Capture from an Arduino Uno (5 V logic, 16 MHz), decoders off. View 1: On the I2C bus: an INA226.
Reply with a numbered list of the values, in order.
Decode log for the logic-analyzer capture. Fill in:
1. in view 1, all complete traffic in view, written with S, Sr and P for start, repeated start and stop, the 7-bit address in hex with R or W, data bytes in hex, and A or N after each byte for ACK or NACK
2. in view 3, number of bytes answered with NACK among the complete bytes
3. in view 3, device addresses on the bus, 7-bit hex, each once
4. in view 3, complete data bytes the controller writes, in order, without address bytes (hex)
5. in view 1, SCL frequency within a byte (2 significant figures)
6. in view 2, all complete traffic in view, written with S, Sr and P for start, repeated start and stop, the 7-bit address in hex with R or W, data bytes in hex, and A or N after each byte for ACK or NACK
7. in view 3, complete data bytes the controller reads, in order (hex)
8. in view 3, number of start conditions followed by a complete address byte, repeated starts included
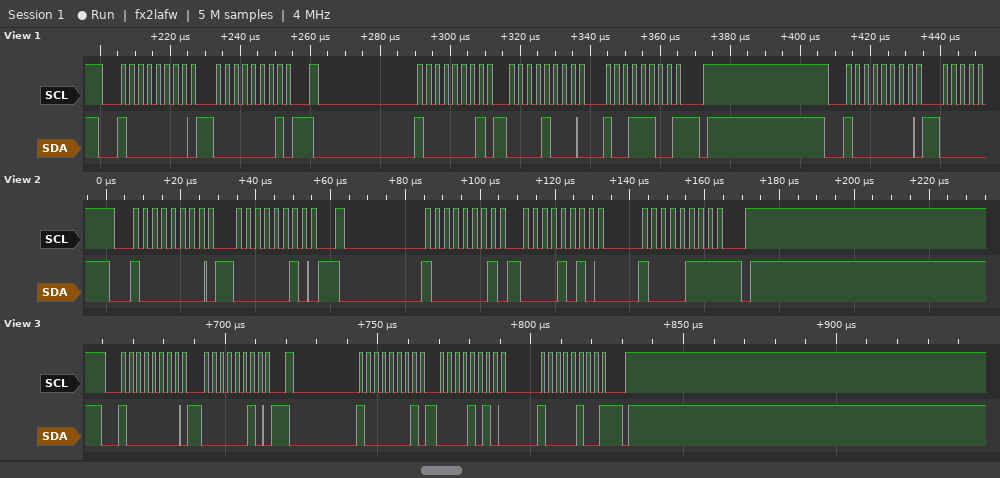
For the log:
1. S 40W A 01 A Sr 40R A 08 A 9C N P S 40W A
2. 1
3. 0x40
4. 02
5. 400 kHz
6. S 40W A 02 A Sr 40R A 0A A 87 N P
7. 0A 84
8. 2
